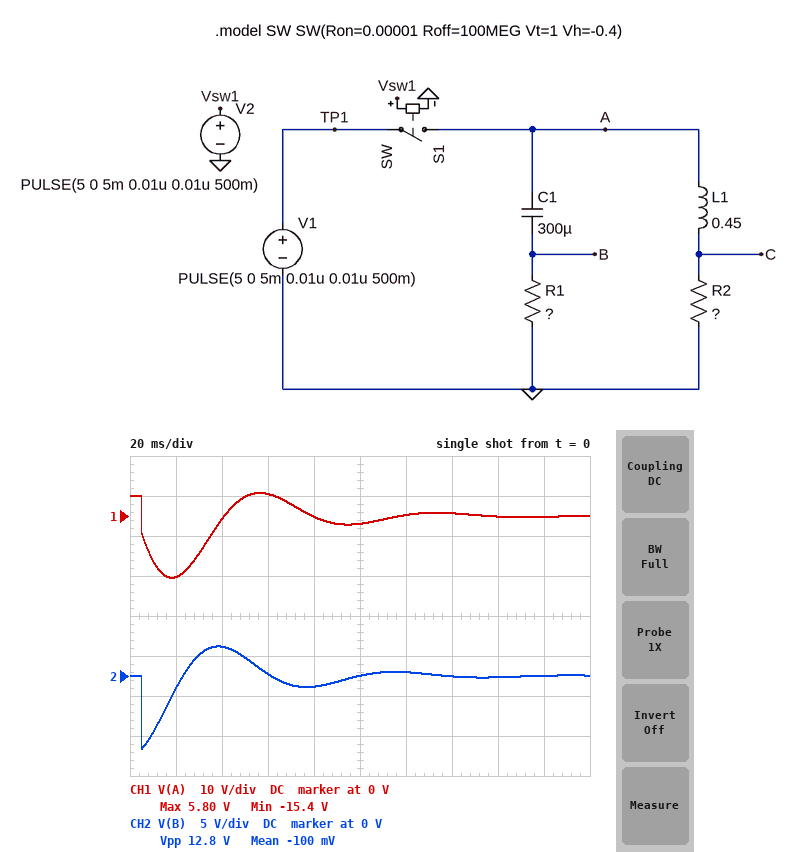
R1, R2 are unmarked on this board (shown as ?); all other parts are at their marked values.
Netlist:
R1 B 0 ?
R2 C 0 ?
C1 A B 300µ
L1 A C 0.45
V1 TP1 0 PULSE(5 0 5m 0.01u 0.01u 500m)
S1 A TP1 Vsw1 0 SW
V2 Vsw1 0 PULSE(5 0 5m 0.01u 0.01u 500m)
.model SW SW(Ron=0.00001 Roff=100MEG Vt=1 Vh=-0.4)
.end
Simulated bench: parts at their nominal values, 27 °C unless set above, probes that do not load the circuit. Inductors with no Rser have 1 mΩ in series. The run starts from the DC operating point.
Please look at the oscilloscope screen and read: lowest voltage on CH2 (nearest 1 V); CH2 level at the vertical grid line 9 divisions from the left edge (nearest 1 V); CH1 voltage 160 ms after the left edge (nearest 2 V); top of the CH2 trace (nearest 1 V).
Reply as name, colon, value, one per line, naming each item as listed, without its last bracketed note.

lowest voltage on CH2: -9 V
CH2 level at the vertical grid line 9 divisions from the left edge: 0 V
CH1 voltage 160 ms after the left edge: 0 V
top of the CH2 trace: 4 V
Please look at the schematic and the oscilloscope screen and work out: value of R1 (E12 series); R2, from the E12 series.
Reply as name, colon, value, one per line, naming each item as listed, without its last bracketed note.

value of R1: 15 Ω
R2, from the E12 series: 8.2 Ω
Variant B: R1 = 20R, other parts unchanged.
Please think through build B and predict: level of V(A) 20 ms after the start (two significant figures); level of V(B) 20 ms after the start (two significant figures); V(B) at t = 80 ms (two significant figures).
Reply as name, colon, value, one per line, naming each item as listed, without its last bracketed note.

level of V(A) 20 ms after the start: -14 V
level of V(B) 20 ms after the start: -1.6 V
V(B) at t = 80 ms: -1.2 V
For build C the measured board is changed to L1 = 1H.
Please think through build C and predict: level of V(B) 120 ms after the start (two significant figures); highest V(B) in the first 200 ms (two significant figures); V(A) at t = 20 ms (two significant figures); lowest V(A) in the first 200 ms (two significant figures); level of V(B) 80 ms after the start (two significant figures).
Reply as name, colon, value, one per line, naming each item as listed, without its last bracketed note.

level of V(B) 120 ms after the start: -2.3 V
highest V(B) in the first 200 ms: 5.0 V
V(A) at t = 20 ms: -24 V
lowest V(A) in the first 200 ms: -26 V
level of V(B) 80 ms after the start: 1.5 V
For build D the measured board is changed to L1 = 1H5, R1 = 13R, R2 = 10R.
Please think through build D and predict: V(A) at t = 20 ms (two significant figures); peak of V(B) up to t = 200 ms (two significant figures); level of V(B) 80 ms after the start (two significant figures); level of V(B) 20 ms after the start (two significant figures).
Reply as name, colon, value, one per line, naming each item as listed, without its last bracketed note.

V(A) at t = 20 ms: -21 V
peak of V(B) up to t = 200 ms: 3.9 V
level of V(B) 80 ms after the start: 3.4 V
level of V(B) 20 ms after the start: -4.4 V
